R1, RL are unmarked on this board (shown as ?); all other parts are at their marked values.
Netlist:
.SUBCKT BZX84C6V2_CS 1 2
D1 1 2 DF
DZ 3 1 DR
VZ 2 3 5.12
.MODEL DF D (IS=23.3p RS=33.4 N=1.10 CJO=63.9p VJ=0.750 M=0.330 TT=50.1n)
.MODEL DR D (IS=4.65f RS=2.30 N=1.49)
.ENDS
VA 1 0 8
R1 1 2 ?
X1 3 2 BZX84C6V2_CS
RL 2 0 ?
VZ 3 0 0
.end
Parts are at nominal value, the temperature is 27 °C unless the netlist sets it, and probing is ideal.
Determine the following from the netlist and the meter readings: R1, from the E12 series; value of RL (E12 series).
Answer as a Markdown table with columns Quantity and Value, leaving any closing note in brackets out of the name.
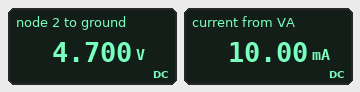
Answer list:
| Quantity | Value |
|---|---|
| R1, from the E12 series | 330 Ω |
| value of RL | 470 Ω |
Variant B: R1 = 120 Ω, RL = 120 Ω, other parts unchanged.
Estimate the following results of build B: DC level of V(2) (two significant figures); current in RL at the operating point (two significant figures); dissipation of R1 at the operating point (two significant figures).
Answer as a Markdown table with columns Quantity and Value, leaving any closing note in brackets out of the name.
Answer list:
| Quantity | Value |
|---|---|
| DC level of V(2) | 4.0 V |
| current in RL at the operating point | 33 mA |
| dissipation of R1 at the operating point | 130 mW |
